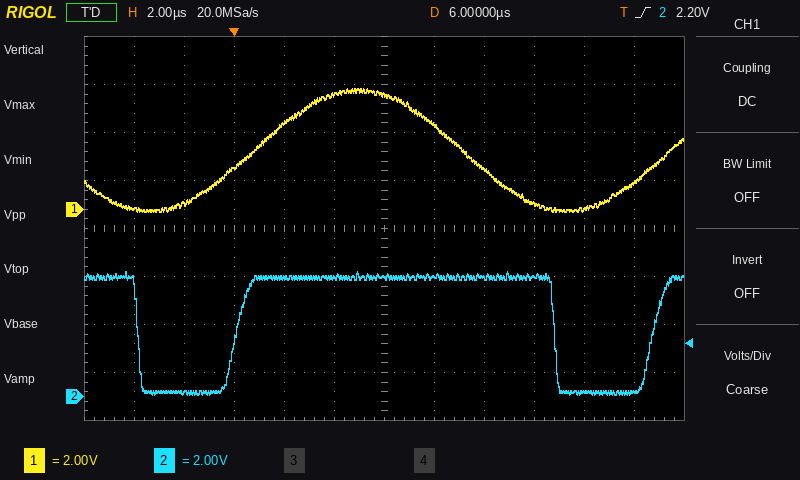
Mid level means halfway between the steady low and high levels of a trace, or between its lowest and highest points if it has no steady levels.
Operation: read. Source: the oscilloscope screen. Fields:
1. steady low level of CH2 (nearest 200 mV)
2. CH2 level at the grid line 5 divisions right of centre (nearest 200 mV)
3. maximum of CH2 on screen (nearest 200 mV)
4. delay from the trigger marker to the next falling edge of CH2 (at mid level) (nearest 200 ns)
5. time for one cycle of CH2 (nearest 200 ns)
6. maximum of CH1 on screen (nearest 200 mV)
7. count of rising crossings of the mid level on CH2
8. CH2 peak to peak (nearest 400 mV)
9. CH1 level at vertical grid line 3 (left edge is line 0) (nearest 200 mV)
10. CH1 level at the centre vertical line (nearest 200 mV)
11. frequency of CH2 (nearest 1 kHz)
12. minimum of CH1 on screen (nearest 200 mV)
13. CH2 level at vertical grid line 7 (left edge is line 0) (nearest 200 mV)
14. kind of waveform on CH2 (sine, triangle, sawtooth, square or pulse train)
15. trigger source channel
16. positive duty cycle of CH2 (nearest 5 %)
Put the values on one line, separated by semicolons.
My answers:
200 mV; 200 mV; 5.2 V; 12.8 µs; 16.6 µs; 5.0 V; 2; 5.2 V; 1.8 V; 4.8 V; 60 kHz; 0.0 V; 5.0 V; pulse train; CH2; 75 %
